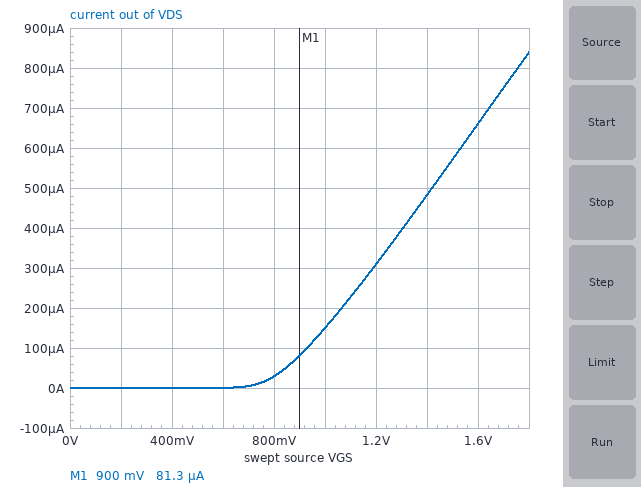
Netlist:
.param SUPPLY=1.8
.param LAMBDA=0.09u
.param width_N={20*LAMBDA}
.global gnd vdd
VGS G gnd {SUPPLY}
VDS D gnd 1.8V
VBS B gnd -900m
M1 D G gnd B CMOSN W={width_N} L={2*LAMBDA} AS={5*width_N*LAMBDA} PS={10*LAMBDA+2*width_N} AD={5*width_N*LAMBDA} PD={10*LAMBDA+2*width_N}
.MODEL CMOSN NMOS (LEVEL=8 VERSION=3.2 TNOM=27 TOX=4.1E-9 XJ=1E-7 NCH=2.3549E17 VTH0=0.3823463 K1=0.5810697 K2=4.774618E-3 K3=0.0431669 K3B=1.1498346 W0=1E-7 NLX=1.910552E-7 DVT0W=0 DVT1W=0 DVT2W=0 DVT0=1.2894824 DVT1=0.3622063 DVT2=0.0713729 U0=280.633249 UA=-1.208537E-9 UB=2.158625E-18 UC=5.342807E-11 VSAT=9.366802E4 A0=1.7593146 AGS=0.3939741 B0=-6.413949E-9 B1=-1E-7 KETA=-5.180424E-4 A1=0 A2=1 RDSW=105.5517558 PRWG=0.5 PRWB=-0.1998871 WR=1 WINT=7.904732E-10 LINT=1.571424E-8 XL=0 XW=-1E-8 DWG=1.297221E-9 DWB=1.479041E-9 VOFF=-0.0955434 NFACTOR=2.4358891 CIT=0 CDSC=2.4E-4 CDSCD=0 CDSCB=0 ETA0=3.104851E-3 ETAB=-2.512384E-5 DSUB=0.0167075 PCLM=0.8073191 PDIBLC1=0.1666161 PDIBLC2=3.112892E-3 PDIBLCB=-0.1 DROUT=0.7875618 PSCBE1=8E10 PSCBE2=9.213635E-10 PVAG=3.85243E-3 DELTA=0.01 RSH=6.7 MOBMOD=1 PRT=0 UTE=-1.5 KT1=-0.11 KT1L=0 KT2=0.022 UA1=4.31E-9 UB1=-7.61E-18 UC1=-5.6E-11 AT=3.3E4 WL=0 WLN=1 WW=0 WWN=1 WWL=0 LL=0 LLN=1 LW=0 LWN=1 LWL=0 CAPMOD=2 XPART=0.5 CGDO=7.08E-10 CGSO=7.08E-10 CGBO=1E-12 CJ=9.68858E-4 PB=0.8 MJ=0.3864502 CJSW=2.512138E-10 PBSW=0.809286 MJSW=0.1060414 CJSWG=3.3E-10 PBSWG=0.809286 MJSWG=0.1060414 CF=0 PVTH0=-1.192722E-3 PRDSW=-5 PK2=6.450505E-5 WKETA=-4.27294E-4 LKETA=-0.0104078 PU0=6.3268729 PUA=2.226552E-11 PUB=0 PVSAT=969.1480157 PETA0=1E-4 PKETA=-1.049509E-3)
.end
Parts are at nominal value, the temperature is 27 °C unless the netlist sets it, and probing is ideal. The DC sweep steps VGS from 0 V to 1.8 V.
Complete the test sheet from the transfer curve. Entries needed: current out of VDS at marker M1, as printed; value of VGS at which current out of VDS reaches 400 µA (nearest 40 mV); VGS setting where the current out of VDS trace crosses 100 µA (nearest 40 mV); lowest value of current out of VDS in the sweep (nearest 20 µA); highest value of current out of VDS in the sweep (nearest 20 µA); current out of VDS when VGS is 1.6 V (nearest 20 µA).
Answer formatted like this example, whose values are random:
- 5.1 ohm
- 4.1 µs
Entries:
- 81.3 µA
- 1.32 V
- 920 mV
- 0 A
- 840 µA
- 660 µA
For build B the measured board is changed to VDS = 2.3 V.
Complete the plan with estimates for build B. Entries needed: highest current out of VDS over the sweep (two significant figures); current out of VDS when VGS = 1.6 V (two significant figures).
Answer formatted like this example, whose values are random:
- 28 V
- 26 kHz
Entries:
- 860 µA
- 680 µA
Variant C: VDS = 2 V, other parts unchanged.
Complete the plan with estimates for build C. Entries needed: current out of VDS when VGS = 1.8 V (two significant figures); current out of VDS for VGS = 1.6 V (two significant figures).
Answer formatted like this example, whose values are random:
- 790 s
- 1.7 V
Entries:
- 850 µA
- 670 µA
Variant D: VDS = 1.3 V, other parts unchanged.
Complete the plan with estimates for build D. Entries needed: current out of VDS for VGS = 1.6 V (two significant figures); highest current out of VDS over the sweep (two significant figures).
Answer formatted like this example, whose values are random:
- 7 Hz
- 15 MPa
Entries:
- 640 µA
- 810 µA
